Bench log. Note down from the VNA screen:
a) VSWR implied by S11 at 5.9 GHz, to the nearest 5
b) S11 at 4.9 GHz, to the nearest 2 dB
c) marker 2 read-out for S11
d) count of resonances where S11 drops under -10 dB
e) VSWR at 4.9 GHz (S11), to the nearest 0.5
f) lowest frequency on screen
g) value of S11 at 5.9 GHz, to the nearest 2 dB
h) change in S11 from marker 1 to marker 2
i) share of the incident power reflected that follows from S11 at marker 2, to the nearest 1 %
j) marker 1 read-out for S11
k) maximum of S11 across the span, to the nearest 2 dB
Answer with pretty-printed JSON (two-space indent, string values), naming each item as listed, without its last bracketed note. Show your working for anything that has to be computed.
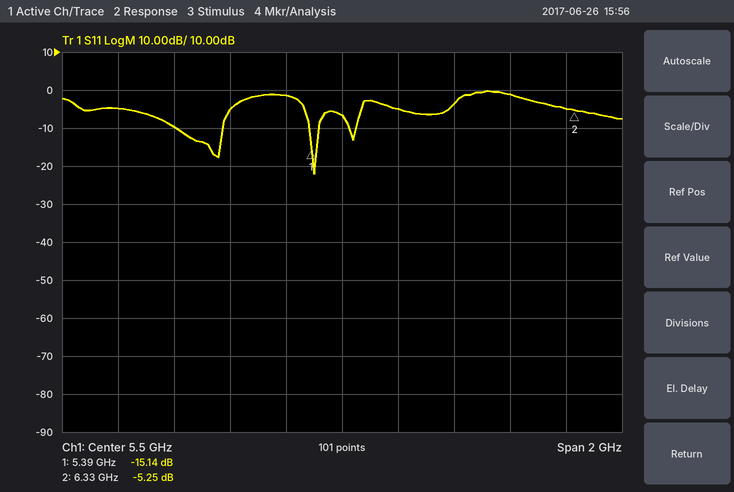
{
  "VSWR implied by S11 at 5.9 GHz, to the nearest 5": "|Γ| = 10^(-4/20) = 0.6310; VSWR = (1 + 0.6310)/(1 − 0.6310) ≈ 4.42, so 5 to the nearest 5",
  "S11 at 4.9 GHz, to the nearest 2 dB": "-10 dB",
  "marker 2 read-out for S11": "-5.25 dB",
  "count of resonances where S11 drops under -10 dB": "3",
  "VSWR at 4.9 GHz (S11), to the nearest 0.5": "|Γ| = 10^(-10/20) = 0.3162; VSWR = (1 + 0.3162)/(1 − 0.3162) ≈ 1.92, so 2.0 to the nearest 0.5",
  "lowest frequency on screen": "4.5 GHz",
  "value of S11 at 5.9 GHz, to the nearest 2 dB": "-4 dB",
  "change in S11 from marker 1 to marker 2": "-5.25 − (-15.14) = 9.89 dB",
  "share of the incident power reflected that follows from S11 at marker 2, to the nearest 1 %": "10^(-5.25/10) ≈ 30 %",
  "marker 1 read-out for S11": "-15.14 dB",
  "maximum of S11 across the span, to the nearest 2 dB": "0 dB"
}
